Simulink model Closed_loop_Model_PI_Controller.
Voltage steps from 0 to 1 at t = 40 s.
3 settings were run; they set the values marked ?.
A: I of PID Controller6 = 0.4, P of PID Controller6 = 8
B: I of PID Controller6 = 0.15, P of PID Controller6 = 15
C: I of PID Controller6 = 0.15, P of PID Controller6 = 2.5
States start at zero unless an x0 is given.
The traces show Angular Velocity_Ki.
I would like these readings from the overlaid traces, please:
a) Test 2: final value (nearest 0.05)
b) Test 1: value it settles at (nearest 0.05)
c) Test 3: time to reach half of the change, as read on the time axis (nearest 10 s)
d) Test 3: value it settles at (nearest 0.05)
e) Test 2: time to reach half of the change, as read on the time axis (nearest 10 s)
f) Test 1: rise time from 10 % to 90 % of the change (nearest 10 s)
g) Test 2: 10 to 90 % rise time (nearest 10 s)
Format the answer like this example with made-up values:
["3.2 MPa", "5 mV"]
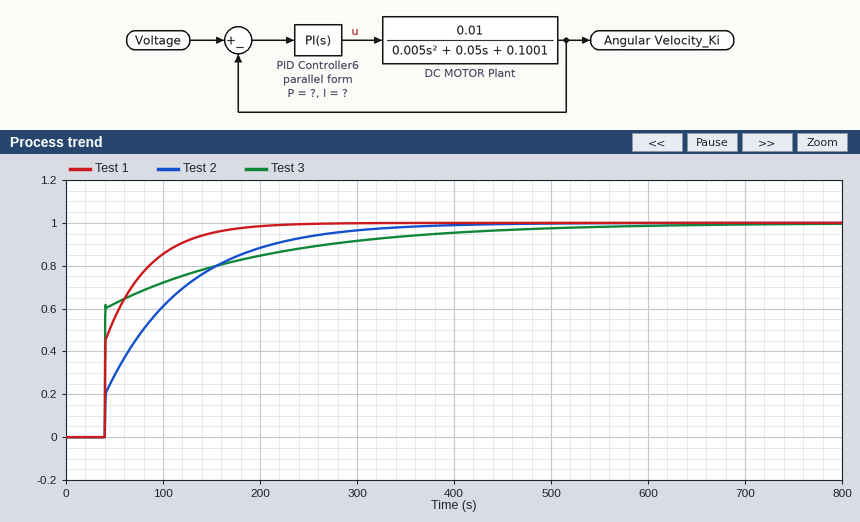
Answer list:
["1.00", "1.00", "40 s", "1.00", "80 s", "80 s", "170 s"]
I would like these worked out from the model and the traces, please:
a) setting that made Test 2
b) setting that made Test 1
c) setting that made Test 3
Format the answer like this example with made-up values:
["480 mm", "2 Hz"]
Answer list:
["C", "A", "B"]
